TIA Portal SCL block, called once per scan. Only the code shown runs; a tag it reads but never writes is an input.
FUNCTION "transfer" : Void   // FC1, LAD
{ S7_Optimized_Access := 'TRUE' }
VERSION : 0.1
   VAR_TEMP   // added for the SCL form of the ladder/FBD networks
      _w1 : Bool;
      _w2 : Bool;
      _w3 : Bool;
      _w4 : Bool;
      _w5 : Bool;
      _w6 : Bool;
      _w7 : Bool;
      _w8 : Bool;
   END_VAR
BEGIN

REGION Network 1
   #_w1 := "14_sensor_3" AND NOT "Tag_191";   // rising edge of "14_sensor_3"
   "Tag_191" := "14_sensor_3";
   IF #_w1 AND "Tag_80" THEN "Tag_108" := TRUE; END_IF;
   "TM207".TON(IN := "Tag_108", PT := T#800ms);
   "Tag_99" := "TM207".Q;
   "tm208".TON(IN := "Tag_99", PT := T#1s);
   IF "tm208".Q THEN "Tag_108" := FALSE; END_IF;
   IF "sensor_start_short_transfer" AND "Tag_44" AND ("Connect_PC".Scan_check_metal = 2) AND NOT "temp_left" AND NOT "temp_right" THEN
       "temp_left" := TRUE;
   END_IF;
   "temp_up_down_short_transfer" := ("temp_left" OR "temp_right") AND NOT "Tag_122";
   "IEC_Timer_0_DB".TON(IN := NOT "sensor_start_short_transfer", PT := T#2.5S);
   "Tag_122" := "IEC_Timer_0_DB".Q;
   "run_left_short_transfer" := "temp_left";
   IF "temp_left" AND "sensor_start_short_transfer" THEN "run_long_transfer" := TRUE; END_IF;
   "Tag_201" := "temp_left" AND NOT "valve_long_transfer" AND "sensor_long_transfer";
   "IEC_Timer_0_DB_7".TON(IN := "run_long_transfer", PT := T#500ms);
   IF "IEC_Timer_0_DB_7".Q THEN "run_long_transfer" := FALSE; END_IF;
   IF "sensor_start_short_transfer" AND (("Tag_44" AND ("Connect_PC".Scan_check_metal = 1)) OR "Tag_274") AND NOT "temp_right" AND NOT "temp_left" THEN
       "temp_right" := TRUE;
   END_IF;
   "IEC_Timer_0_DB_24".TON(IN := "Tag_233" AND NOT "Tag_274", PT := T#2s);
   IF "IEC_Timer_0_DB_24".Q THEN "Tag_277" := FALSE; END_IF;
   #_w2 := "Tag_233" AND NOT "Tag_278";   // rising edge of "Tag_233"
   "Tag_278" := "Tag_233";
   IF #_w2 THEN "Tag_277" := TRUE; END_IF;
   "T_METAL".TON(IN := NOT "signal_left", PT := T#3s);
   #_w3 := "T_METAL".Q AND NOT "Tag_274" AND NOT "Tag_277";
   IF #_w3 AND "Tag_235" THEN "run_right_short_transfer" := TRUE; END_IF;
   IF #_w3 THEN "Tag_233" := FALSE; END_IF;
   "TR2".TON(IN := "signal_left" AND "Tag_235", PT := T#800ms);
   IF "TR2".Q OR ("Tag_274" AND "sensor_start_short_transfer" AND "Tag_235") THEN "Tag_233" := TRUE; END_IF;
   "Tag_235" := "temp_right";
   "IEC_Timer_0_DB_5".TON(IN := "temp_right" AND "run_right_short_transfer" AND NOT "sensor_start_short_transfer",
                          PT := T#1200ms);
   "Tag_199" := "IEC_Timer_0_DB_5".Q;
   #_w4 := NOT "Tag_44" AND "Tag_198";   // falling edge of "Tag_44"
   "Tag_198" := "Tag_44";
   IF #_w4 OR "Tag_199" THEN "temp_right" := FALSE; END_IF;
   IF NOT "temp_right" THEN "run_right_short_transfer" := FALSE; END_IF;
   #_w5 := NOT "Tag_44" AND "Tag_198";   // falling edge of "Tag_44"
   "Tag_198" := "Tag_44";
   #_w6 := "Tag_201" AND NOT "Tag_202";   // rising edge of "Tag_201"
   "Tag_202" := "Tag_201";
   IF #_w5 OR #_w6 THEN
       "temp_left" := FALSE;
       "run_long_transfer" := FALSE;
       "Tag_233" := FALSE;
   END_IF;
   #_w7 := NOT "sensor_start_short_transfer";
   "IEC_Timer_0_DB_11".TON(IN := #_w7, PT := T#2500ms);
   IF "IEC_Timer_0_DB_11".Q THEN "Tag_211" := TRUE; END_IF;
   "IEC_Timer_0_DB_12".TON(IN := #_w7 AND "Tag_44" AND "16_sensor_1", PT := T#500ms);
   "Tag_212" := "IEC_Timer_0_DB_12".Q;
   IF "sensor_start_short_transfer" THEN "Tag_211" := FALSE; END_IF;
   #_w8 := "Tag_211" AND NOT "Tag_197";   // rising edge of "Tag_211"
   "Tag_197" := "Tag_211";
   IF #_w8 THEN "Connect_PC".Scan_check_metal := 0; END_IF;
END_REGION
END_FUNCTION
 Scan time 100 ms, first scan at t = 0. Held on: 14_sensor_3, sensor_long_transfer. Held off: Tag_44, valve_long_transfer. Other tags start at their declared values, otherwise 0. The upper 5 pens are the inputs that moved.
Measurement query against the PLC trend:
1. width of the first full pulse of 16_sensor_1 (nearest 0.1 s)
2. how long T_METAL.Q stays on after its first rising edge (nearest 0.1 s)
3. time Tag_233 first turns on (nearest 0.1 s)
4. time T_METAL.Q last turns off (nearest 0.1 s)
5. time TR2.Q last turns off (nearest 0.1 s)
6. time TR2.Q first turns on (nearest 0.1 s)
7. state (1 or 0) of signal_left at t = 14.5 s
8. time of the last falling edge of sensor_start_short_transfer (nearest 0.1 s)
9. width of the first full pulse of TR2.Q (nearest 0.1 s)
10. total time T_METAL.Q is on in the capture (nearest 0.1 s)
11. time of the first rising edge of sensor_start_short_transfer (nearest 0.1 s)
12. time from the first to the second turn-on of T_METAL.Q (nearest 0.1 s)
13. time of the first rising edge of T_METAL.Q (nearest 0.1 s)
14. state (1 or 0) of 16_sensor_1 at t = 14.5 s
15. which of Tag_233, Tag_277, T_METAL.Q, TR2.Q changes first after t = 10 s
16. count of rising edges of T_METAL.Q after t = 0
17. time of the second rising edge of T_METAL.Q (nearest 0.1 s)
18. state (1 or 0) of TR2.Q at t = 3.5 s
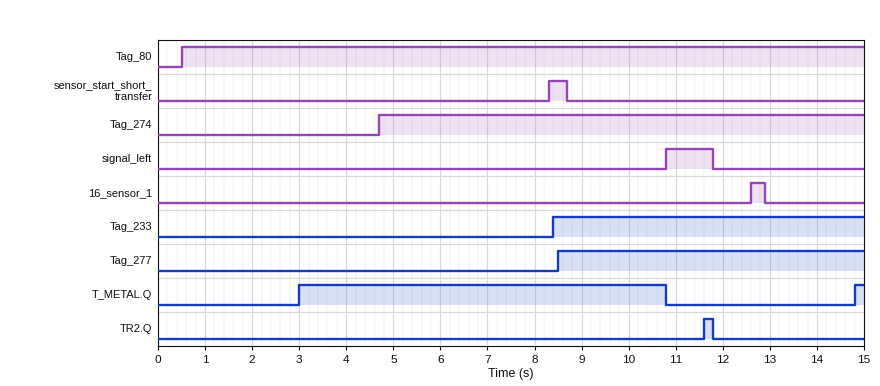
0.3 s
7.8 s
8.4 s
10.8 s
11.8 s
11.6 s
0
8.7 s
0.2 s
8.0 s
8.3 s
11.8 s
3.0 s
0
T_METAL.Q
2
14.8 s
0
